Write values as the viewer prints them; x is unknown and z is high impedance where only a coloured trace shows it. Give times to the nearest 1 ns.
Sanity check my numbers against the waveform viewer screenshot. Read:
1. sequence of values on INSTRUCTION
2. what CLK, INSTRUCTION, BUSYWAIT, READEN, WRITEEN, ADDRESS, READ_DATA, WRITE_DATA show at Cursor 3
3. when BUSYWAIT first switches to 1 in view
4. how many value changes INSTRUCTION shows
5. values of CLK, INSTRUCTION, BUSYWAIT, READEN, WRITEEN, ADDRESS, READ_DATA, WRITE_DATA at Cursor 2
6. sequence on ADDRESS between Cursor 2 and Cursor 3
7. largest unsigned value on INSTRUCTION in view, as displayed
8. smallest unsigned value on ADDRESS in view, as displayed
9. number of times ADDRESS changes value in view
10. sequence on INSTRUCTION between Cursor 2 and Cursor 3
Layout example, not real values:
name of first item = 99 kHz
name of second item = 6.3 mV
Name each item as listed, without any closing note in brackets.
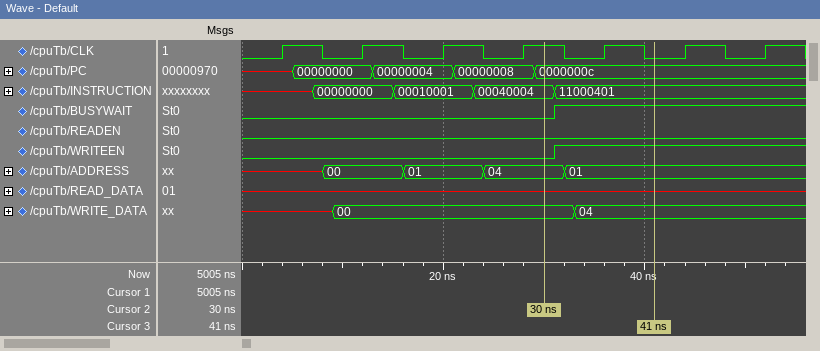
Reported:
sequence of values on INSTRUCTION = x, 00000000, 00010001, 00040004, 11000401
what CLK, INSTRUCTION, BUSYWAIT, READEN, WRITEEN, ADDRESS, READ_DATA, WRITE_DATA show at Cursor 3 = CLK=0, INSTRUCTION=11000401, BUSYWAIT=1, READEN=0, WRITEEN=1, ADDRESS=01, READ_DATA=x, WRITE_DATA=04
when BUSYWAIT first switches to 1 in view = 31 ns
how many value changes INSTRUCTION shows = 4
values of CLK, INSTRUCTION, BUSYWAIT, READEN, WRITEEN, ADDRESS, READ_DATA, WRITE_DATA at Cursor 2 = CLK=1, INSTRUCTION=00040004, BUSYWAIT=0, READEN=0, WRITEEN=0, ADDRESS=04, READ_DATA=x, WRITE_DATA=00
sequence on ADDRESS between Cursor 2 and Cursor 3 = 04, 01
largest unsigned value on INSTRUCTION in view, as displayed = 11000401
smallest unsigned value on ADDRESS in view, as displayed = 00
number of times ADDRESS changes value in view = 4
sequence on INSTRUCTION between Cursor 2 and Cursor 3 = 00040004, 11000401
